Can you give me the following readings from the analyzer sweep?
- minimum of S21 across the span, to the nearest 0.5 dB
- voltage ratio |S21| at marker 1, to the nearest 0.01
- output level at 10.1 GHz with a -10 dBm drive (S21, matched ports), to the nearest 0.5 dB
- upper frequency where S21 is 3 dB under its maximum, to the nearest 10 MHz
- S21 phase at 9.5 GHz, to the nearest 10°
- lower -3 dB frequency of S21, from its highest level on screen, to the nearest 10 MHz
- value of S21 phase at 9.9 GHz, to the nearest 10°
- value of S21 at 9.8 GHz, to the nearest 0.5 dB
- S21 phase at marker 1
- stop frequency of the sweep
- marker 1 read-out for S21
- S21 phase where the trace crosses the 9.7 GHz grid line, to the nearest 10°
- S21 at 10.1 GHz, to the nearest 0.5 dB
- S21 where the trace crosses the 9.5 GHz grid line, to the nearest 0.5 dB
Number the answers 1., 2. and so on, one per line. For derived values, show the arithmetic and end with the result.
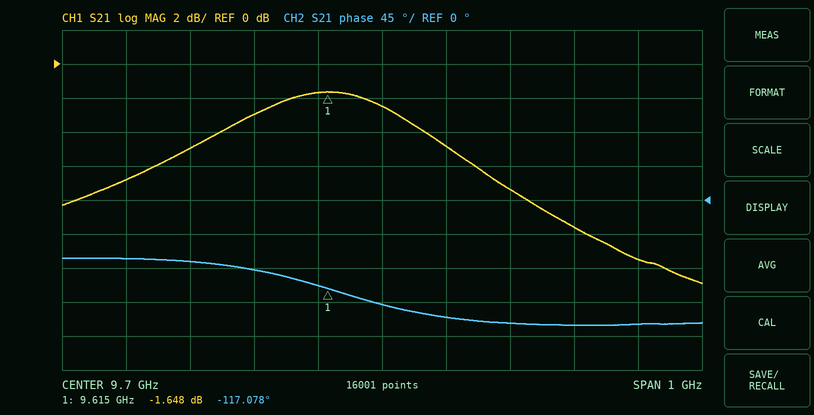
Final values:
1. -13.0 dB
2. 10^(-1.648/20) ≈ 0.83
3. -10 dBm + (-11.5 dB) = -21.5 dBm
4. 9.79 GHz
5. -90°
6. 9.42 GHz
7. -160°
8. -5.0 dB
9. -117.078°
10. 10.2 GHz
11. -1.648 dB
12. -140°
13. -11.5 dB
14. -3.0 dB
